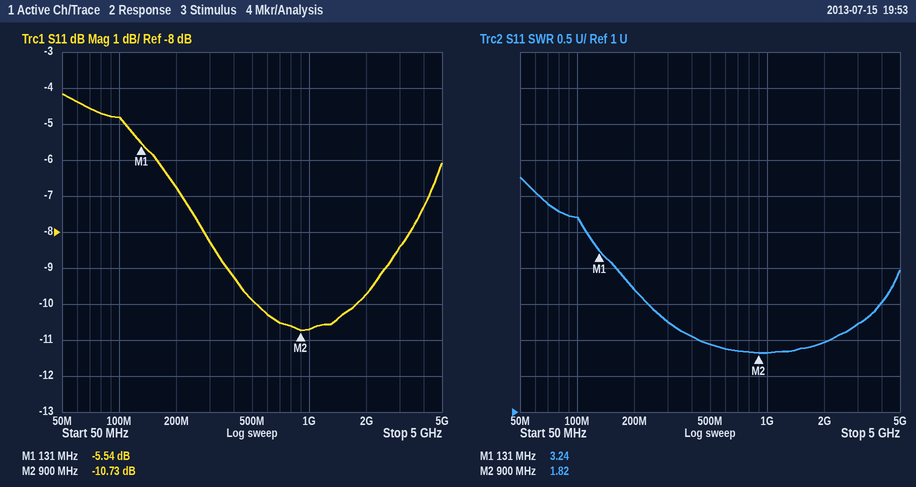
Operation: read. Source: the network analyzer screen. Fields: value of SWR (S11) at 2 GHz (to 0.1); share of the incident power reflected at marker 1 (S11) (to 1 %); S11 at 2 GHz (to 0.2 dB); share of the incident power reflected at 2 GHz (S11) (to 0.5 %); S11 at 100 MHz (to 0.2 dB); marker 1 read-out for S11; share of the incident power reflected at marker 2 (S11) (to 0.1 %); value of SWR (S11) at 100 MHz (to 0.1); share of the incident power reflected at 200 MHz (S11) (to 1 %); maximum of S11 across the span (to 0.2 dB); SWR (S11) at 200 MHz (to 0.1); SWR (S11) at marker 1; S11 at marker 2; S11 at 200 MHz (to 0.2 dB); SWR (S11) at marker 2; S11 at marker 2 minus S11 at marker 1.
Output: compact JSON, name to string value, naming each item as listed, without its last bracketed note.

{"value of SWR (S11) at 2 GHz": "2.0", "share of the incident power reflected at marker 1 (S11)": "28 %", "S11 at 2 GHz": "-9.8 dB", "share of the incident power reflected at 2 GHz (S11)": "10.5 %", "S11 at 100 MHz": "-4.8 dB", "marker 1 read-out for S11": "-5.54 dB", "share of the incident power reflected at marker 2 (S11)": "8.5 %", "value of SWR (S11) at 100 MHz": "3.7", "share of the incident power reflected at 200 MHz (S11)": "21 %", "maximum of S11 across the span": "-4.2 dB", "SWR (S11) at 200 MHz": "2.7", "SWR (S11) at marker 1": "3.24", "S11 at marker 2": "-10.73 dB", "S11 at 200 MHz": "-6.8 dB", "SWR (S11) at marker 2": "1.82", "S11 at marker 2 minus S11 at marker 1": "-5.19 dB"}
